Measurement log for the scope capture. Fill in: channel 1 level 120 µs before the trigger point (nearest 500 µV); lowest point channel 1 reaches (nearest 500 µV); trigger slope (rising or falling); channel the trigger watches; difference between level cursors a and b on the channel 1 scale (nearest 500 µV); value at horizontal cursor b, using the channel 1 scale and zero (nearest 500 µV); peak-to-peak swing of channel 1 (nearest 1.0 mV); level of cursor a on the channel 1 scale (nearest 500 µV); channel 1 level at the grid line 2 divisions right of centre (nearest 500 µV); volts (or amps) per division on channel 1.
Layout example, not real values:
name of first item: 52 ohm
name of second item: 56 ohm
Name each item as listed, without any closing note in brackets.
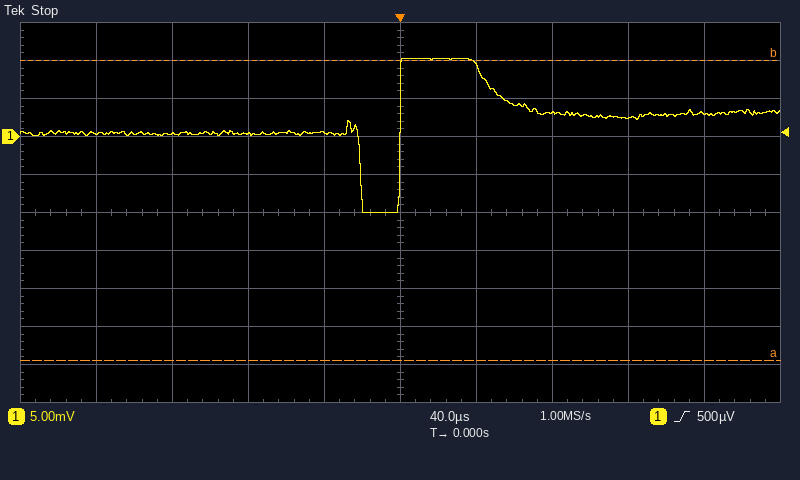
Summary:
channel 1 level 120 µs before the trigger point: 500 µV
lowest point channel 1 reaches: -10.0 mV
trigger slope: rising
channel the trigger watches: channel 1
difference between level cursors a and b on the channel 1 scale: 39.5 mV
value at horizontal cursor b, using the channel 1 scale and zero: 10.0 mV
peak-to-peak swing of channel 1: 20.0 mV
level of cursor a on the channel 1 scale: -29.5 mV
channel 1 level at the grid line 2 divisions right of centre: 3.0 mV
volts (or amps) per division on channel 1: 5 mV
